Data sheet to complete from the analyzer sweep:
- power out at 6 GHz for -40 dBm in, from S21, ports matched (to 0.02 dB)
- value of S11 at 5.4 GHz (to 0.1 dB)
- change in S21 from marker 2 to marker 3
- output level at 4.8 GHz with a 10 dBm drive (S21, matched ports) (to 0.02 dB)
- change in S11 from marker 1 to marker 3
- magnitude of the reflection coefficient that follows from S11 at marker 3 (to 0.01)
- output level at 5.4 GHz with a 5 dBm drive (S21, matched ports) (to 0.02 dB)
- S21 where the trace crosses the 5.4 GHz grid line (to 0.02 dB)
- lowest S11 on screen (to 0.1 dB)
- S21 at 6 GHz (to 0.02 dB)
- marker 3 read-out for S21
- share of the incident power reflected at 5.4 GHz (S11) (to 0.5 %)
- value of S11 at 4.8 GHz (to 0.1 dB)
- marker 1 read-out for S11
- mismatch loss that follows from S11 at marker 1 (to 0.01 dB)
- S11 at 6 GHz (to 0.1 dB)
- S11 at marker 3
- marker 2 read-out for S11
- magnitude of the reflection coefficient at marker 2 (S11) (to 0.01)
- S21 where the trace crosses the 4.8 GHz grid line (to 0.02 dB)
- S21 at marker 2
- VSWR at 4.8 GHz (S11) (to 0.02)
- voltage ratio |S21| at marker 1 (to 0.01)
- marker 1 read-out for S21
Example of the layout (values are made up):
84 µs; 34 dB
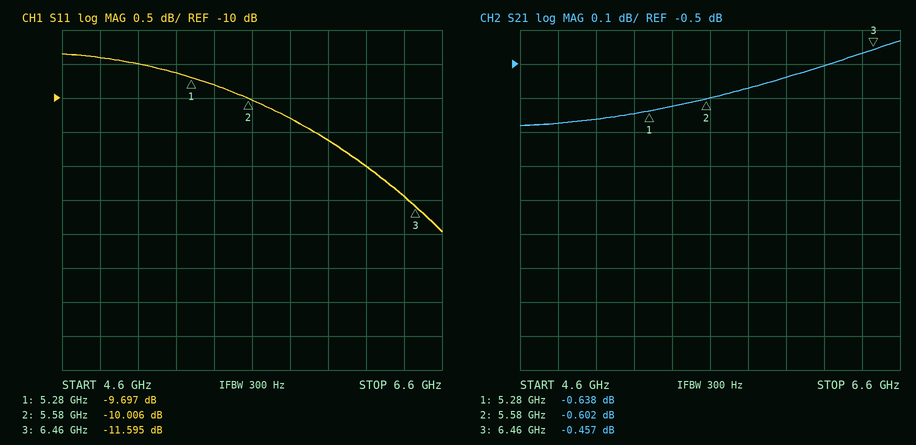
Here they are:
-40.54 dBm; -9.8 dB; 0.145 dB; 9.32 dBm; -1.898 dB; 0.26; 4.38 dBm; -0.62 dB; -12.0 dB; -0.54 dB; -0.457 dB; 10.5 %; -9.4 dB; -9.697 dB; 0.49 dB; -10.6 dB; -11.595 dB; -10.006 dB; 0.32; -0.68 dB; -0.602 dB; 2.02; 0.93; -0.638 dB
